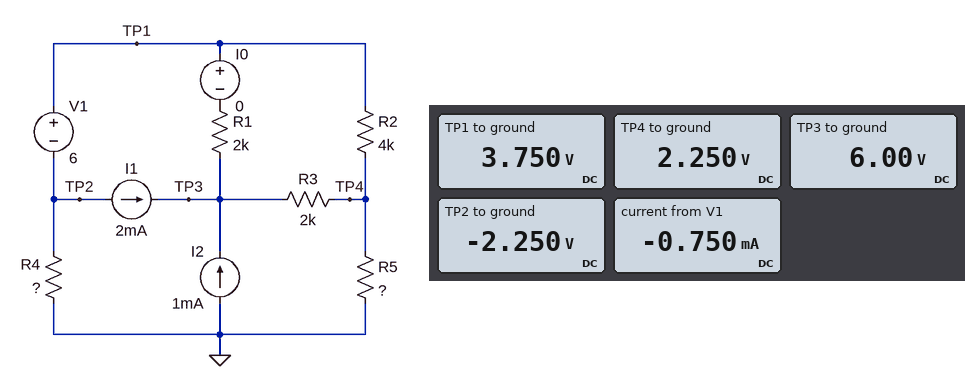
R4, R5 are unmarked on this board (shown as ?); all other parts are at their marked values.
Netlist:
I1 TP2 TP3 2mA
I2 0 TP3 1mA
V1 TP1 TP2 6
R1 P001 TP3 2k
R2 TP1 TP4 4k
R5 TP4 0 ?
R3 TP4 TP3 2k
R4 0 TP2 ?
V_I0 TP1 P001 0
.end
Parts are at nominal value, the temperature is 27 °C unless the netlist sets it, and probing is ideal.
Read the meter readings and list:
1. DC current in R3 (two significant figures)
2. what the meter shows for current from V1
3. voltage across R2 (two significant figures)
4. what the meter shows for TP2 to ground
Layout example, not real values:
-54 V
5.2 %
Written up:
1.9 mA
-0.750 mA
1.5 V
-2.250 V
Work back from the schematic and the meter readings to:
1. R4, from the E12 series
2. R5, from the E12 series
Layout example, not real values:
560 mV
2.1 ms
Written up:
1.8 kΩ
1 kΩ
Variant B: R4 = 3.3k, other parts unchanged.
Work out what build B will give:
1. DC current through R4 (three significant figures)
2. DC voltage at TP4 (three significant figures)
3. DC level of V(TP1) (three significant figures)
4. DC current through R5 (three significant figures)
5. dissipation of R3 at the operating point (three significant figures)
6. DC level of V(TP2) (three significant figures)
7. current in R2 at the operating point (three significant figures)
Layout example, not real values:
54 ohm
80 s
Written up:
952 µA
1.95 V
2.86 V
1.95 mA
5.96 mW
-3.14 V
226 µA
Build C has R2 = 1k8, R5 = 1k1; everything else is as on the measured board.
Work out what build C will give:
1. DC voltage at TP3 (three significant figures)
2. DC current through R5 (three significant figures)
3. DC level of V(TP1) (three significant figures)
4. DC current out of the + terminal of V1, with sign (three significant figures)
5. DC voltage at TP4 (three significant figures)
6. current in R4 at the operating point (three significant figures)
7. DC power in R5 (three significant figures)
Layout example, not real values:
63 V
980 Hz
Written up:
6.08 V
2.33 mA
3.60 V
-667 µA
2.57 V
1.33 mA
5.99 mW
